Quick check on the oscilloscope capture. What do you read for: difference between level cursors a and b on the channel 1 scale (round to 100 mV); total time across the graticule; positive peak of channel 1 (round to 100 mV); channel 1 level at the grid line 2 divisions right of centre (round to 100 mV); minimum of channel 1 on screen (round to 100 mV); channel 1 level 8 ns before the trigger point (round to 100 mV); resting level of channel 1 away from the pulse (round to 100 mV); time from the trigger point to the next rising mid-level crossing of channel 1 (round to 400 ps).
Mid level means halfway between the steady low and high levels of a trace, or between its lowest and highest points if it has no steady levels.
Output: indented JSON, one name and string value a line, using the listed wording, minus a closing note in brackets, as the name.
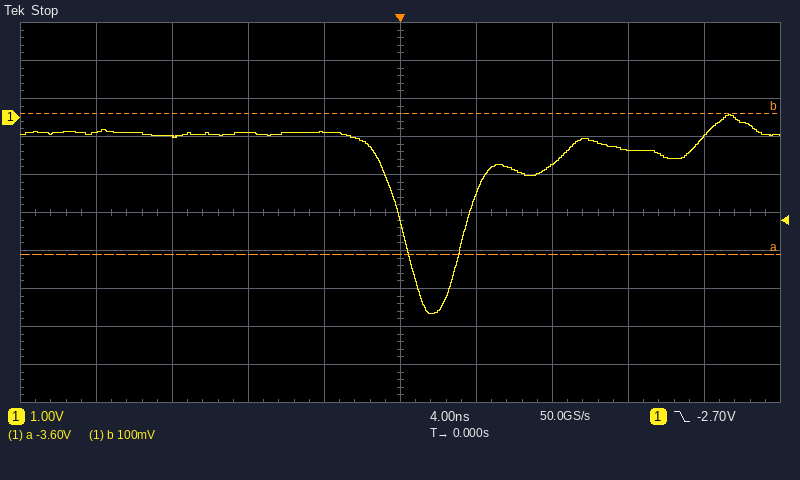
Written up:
{
  "difference between level cursors a and b on the channel 1 scale": "3.7 V",
  "total time across the graticule": "40 ns",
  "positive peak of channel 1": "100 mV",
  "channel 1 level at the grid line 2 divisions right of centre": "-1.2 V",
  "minimum of channel 1 on screen": "-5.2 V",
  "channel 1 level 8 ns before the trigger point": "-400 mV",
  "resting level of channel 1 away from the pulse": "-400 mV",
  "time from the trigger point to the next rising mid-level crossing of channel 1": "3.6 ns"
}
